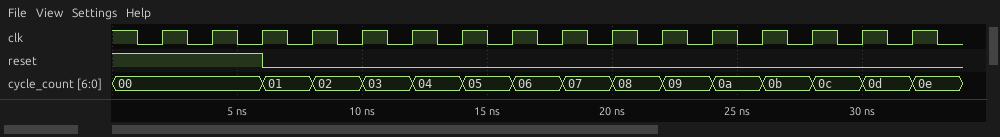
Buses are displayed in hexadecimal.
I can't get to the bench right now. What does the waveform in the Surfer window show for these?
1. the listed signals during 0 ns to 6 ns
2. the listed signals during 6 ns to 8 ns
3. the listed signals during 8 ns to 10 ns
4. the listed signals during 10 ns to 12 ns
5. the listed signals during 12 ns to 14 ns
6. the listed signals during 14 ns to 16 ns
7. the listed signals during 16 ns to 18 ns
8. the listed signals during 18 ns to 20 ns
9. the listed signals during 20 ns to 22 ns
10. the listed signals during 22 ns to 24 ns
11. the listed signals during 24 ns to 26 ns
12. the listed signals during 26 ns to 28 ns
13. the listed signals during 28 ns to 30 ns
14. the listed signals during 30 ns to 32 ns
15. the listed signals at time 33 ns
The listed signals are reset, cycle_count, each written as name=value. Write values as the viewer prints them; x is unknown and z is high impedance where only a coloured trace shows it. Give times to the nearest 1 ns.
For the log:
reset=1, cycle_count=00
reset=0, cycle_count=01
reset=0, cycle_count=02
reset=0, cycle_count=03
reset=0, cycle_count=04
reset=0, cycle_count=05
reset=0, cycle_count=06
reset=0, cycle_count=07
reset=0, cycle_count=08
reset=0, cycle_count=09
reset=0, cycle_count=0a
reset=0, cycle_count=0b
reset=0, cycle_count=0c
reset=0, cycle_count=0d
reset=0, cycle_count=0e
